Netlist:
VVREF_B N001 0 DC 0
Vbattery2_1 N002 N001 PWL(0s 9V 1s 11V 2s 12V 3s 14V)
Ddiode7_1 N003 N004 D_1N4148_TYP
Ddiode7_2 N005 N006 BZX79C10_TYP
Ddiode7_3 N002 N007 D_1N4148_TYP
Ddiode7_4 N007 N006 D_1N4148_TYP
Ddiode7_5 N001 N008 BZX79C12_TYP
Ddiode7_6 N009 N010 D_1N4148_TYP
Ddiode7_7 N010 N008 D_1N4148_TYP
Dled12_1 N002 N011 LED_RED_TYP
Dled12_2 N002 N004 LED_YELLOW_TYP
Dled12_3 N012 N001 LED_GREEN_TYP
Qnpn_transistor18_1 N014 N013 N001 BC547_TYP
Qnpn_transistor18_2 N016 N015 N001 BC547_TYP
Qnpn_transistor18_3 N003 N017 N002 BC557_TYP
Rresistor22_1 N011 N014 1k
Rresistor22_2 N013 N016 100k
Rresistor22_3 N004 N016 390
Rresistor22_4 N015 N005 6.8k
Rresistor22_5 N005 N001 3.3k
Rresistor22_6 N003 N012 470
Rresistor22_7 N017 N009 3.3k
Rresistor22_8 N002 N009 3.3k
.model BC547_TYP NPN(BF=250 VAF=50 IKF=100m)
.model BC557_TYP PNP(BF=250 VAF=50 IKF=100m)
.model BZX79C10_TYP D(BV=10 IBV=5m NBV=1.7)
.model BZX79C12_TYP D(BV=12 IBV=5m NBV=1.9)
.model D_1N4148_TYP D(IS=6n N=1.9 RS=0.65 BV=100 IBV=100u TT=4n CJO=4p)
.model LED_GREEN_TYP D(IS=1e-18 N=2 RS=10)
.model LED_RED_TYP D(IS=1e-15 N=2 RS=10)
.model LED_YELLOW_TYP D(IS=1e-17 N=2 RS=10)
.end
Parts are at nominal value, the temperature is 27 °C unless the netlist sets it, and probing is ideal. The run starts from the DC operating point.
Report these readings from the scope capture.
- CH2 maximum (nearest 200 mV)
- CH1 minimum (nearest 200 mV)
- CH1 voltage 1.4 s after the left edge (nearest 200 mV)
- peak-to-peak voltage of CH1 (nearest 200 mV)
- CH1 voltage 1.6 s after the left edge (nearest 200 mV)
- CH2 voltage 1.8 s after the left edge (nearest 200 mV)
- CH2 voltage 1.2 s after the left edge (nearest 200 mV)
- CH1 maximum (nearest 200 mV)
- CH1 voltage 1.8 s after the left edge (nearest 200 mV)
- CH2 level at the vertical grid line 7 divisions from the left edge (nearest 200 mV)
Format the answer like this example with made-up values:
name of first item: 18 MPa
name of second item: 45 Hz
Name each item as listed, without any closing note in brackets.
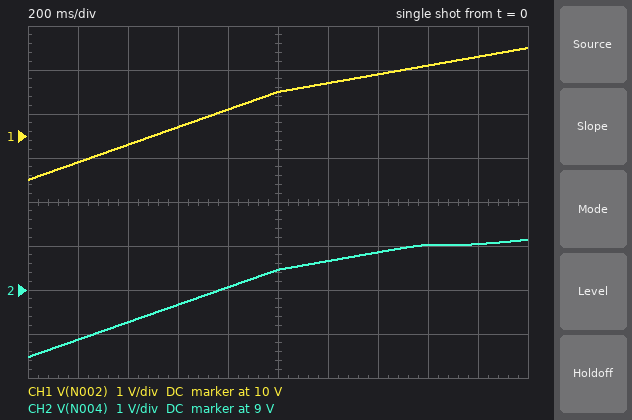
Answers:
CH2 maximum: 10.2 V
CH1 minimum: 9.0 V
CH1 voltage 1.4 s after the left edge: 11.4 V
peak-to-peak voltage of CH1: 3.0 V
CH1 voltage 1.6 s after the left edge: 11.6 V
CH2 voltage 1.8 s after the left edge: 10.0 V
CH2 voltage 1.2 s after the left edge: 9.6 V
CH1 maximum: 12.0 V
CH1 voltage 1.8 s after the left edge: 11.8 V
CH2 level at the vertical grid line 7 divisions from the left edge: 9.8 V
